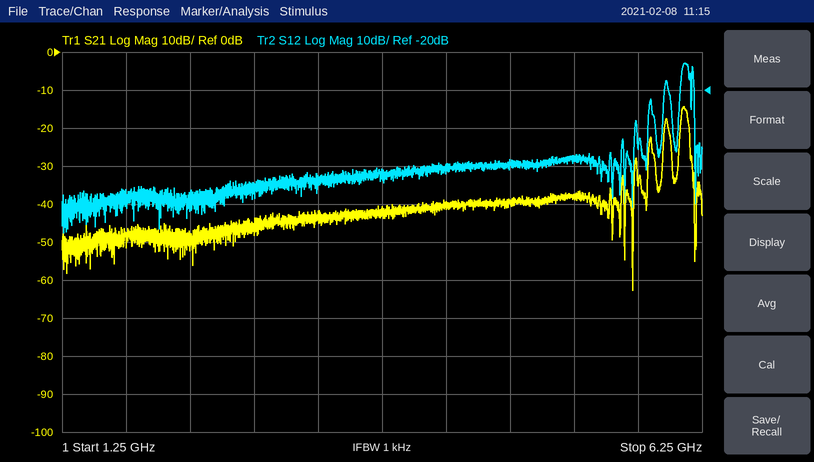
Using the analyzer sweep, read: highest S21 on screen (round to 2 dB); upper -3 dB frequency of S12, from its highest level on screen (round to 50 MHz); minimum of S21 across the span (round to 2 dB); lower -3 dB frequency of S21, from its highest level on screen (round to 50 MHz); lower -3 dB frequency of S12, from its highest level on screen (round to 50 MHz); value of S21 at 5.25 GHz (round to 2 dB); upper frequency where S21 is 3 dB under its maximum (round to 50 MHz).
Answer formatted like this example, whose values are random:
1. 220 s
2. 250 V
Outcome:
1. -14 dB
2. 6.15 GHz
3. -62 dB
4. 6.10 GHz
5. 6.10 GHz
6. -38 dB
7. 6.15 GHz
